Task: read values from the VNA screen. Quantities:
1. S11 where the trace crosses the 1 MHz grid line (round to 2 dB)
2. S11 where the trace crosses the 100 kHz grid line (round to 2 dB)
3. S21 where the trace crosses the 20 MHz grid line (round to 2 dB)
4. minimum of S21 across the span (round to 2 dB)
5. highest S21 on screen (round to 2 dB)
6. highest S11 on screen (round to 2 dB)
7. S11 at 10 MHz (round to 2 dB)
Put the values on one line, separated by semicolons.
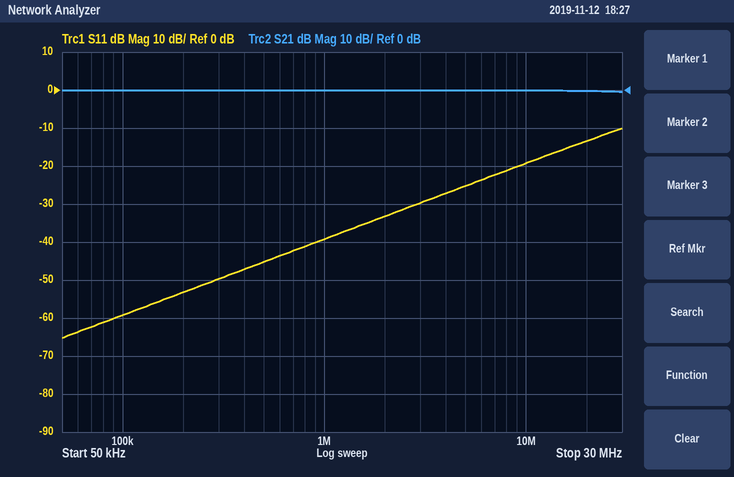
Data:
-40 dB; -60 dB; 0 dB; 0 dB; 0 dB; -10 dB; -20 dB
